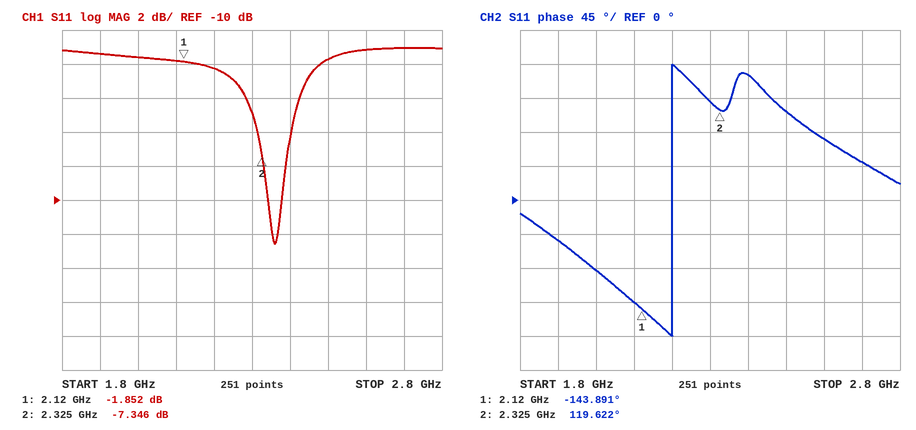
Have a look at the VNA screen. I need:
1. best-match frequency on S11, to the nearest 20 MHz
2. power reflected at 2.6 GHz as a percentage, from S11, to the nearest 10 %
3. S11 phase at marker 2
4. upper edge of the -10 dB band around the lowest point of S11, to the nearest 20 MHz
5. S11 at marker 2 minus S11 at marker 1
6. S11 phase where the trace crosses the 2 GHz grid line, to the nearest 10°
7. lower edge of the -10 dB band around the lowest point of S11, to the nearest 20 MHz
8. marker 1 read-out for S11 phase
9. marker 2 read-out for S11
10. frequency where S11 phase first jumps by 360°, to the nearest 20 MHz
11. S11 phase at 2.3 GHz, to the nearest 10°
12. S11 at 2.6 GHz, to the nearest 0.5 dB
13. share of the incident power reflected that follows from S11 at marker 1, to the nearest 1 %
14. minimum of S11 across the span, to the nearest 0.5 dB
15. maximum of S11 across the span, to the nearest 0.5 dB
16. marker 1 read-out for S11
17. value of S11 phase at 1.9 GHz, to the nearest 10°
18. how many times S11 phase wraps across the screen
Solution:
2.36 GHz
80 %
119.622°
2.38 GHz
-5.494 dB
-90°
2.34 GHz
-143.891°
-7.346 dB
2.20 GHz
130°
-1.0 dB
65 %
-12.5 dB
-1.0 dB
-1.852 dB
-50°
1
